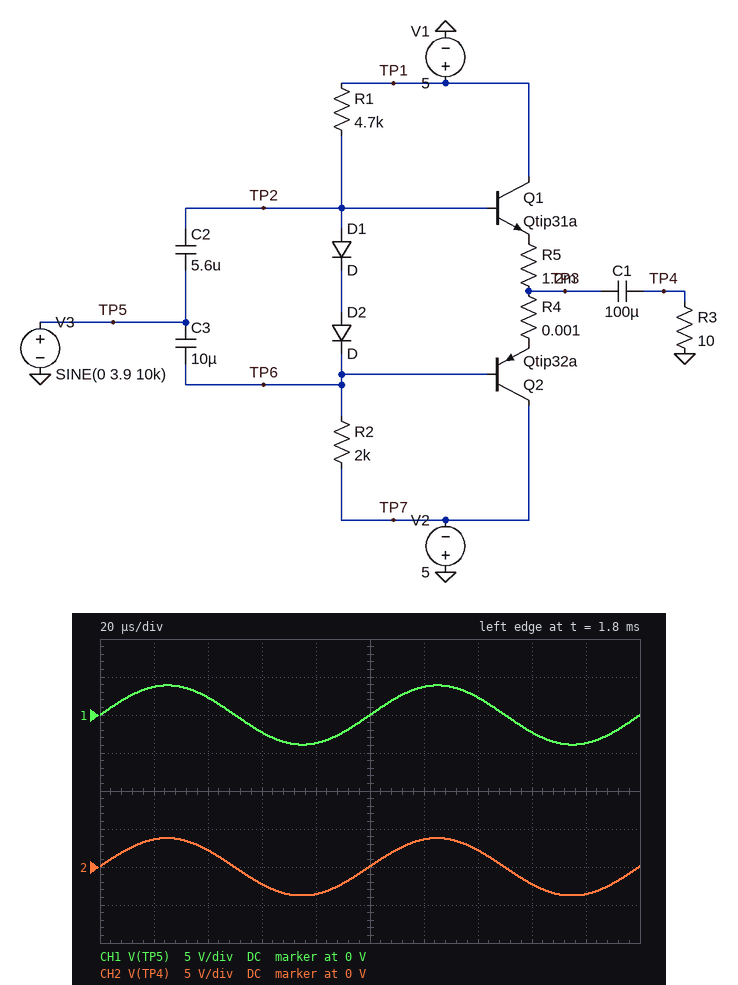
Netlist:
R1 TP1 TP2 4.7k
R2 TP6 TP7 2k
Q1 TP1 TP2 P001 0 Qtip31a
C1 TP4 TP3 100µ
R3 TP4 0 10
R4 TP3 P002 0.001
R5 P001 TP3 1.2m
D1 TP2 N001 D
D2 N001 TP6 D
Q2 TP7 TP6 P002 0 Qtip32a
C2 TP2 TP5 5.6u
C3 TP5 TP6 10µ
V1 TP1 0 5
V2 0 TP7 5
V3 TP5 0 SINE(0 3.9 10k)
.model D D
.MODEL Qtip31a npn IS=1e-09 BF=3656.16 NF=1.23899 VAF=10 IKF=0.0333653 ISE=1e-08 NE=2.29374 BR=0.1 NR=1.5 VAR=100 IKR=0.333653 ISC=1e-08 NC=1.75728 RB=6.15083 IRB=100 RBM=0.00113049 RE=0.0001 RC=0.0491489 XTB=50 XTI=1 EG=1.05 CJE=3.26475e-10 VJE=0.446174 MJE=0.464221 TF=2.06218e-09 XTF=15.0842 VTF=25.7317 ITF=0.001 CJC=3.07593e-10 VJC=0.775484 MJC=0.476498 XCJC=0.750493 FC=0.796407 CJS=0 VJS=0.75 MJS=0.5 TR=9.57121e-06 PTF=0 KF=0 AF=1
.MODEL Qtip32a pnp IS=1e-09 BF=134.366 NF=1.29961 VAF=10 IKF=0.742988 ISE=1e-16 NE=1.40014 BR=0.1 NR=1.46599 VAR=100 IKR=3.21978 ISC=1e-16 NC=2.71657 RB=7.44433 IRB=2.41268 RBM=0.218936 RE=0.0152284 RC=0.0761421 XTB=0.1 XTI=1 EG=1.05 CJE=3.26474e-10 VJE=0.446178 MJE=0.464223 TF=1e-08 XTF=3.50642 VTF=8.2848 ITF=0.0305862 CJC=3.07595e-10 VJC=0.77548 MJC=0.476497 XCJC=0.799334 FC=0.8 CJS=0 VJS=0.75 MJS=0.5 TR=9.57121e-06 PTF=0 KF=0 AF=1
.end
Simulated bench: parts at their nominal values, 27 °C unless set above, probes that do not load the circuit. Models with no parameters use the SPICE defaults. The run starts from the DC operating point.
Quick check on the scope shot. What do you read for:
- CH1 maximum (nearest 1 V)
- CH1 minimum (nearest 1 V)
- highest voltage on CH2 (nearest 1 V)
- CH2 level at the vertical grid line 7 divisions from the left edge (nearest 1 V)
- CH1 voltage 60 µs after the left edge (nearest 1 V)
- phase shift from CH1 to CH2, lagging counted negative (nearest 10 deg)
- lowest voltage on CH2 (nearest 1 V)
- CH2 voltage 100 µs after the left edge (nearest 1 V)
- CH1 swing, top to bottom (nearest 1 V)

4 V
-4 V
4 V
2 V
-2 V
0 deg
-4 V
0 V
8 V
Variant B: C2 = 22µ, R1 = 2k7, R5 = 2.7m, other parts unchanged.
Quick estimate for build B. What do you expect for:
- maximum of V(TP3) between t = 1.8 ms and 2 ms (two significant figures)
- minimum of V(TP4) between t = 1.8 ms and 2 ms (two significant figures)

3.7 V
-3.8 V
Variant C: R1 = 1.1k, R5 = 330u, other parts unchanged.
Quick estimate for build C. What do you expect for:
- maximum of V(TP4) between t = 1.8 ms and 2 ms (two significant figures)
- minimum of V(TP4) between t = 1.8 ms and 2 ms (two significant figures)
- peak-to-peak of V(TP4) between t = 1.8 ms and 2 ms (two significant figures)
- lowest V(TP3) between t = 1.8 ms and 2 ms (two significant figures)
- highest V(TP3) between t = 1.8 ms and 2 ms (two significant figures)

3.6 V
-3.9 V
7.5 V
-2.7 V
4.8 V
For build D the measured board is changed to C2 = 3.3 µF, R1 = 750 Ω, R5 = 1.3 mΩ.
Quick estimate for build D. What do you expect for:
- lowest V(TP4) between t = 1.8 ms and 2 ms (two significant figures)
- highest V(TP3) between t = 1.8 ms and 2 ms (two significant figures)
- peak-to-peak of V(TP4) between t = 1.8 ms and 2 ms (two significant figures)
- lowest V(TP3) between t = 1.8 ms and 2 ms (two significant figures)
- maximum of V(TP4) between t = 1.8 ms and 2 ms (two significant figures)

-3.8 V
4.9 V
7.1 V
-2.3 V
3.3 V
